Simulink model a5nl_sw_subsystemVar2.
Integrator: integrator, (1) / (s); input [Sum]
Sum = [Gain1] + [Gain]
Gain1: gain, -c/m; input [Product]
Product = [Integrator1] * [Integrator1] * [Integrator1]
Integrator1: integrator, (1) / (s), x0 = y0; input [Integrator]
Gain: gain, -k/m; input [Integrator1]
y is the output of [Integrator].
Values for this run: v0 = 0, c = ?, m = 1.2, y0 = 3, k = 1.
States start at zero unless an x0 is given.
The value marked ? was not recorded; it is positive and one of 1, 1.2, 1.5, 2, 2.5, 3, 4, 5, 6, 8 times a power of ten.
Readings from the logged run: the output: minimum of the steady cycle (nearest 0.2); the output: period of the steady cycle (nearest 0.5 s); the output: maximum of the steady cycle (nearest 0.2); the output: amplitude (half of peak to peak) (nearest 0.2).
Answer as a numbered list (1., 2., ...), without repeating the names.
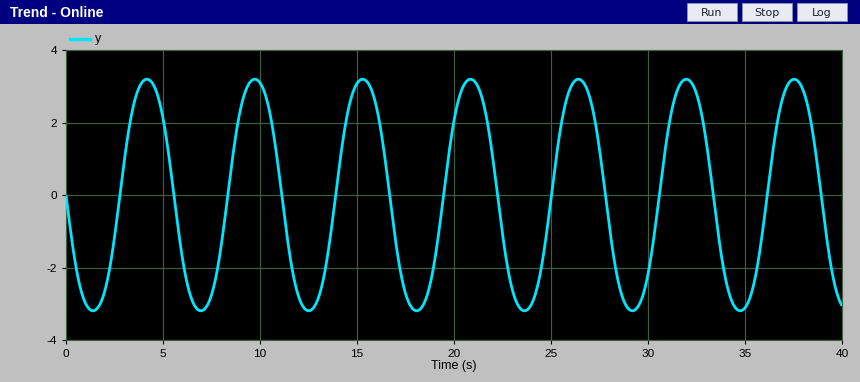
1. -3.2
2. 5.5 s
3. 3.2
4. 3.2
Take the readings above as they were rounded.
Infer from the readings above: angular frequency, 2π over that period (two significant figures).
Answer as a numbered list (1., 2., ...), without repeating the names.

1. 1.1 rad/s
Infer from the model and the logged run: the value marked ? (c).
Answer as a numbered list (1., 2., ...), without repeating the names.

1. 0.08
